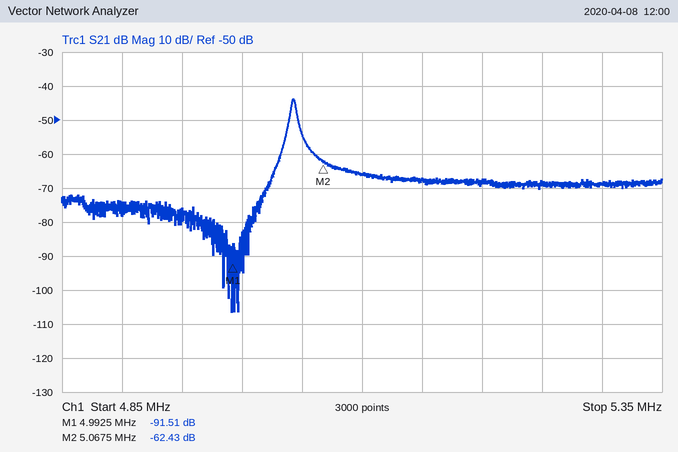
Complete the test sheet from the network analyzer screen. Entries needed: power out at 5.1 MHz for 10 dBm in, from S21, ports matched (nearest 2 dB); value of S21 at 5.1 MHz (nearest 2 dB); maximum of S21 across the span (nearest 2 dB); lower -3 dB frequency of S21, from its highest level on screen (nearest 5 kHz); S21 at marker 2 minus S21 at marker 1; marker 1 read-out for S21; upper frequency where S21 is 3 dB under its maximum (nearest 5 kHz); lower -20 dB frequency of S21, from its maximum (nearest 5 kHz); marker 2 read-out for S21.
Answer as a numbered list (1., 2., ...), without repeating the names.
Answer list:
1. -56 dBm
2. -66 dB
3. -44 dB
4. 5.040 MHz
5. 29.08 dB
6. -91.51 dB
7. 5.045 MHz
8. 5.030 MHz
9. -62.43 dB
